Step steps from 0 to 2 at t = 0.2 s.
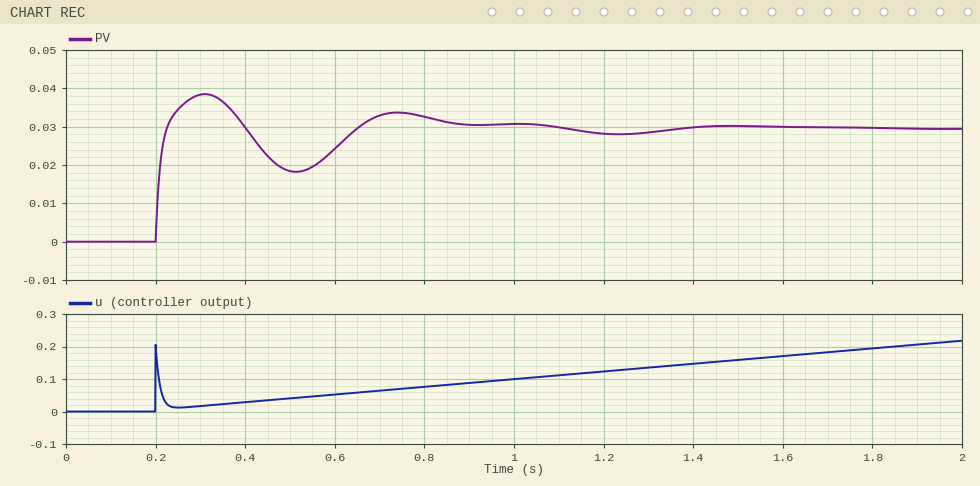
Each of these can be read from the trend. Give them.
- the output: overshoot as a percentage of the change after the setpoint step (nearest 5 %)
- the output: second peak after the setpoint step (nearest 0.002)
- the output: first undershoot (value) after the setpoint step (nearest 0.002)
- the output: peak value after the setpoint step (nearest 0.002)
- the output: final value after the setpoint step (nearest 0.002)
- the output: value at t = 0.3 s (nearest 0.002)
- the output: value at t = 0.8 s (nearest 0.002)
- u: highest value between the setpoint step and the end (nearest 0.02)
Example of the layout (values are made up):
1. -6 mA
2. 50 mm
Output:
1. 30 %
2. 0.034
3. 0.018
4. 0.038
5. 0.030
6. 0.038
7. 0.032
8. 0.22
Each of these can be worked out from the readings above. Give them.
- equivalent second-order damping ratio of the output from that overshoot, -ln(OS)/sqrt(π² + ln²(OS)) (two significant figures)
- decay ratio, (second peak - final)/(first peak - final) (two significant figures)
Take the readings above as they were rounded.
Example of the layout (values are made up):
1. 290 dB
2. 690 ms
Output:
1. 0.36
2. 0.50
